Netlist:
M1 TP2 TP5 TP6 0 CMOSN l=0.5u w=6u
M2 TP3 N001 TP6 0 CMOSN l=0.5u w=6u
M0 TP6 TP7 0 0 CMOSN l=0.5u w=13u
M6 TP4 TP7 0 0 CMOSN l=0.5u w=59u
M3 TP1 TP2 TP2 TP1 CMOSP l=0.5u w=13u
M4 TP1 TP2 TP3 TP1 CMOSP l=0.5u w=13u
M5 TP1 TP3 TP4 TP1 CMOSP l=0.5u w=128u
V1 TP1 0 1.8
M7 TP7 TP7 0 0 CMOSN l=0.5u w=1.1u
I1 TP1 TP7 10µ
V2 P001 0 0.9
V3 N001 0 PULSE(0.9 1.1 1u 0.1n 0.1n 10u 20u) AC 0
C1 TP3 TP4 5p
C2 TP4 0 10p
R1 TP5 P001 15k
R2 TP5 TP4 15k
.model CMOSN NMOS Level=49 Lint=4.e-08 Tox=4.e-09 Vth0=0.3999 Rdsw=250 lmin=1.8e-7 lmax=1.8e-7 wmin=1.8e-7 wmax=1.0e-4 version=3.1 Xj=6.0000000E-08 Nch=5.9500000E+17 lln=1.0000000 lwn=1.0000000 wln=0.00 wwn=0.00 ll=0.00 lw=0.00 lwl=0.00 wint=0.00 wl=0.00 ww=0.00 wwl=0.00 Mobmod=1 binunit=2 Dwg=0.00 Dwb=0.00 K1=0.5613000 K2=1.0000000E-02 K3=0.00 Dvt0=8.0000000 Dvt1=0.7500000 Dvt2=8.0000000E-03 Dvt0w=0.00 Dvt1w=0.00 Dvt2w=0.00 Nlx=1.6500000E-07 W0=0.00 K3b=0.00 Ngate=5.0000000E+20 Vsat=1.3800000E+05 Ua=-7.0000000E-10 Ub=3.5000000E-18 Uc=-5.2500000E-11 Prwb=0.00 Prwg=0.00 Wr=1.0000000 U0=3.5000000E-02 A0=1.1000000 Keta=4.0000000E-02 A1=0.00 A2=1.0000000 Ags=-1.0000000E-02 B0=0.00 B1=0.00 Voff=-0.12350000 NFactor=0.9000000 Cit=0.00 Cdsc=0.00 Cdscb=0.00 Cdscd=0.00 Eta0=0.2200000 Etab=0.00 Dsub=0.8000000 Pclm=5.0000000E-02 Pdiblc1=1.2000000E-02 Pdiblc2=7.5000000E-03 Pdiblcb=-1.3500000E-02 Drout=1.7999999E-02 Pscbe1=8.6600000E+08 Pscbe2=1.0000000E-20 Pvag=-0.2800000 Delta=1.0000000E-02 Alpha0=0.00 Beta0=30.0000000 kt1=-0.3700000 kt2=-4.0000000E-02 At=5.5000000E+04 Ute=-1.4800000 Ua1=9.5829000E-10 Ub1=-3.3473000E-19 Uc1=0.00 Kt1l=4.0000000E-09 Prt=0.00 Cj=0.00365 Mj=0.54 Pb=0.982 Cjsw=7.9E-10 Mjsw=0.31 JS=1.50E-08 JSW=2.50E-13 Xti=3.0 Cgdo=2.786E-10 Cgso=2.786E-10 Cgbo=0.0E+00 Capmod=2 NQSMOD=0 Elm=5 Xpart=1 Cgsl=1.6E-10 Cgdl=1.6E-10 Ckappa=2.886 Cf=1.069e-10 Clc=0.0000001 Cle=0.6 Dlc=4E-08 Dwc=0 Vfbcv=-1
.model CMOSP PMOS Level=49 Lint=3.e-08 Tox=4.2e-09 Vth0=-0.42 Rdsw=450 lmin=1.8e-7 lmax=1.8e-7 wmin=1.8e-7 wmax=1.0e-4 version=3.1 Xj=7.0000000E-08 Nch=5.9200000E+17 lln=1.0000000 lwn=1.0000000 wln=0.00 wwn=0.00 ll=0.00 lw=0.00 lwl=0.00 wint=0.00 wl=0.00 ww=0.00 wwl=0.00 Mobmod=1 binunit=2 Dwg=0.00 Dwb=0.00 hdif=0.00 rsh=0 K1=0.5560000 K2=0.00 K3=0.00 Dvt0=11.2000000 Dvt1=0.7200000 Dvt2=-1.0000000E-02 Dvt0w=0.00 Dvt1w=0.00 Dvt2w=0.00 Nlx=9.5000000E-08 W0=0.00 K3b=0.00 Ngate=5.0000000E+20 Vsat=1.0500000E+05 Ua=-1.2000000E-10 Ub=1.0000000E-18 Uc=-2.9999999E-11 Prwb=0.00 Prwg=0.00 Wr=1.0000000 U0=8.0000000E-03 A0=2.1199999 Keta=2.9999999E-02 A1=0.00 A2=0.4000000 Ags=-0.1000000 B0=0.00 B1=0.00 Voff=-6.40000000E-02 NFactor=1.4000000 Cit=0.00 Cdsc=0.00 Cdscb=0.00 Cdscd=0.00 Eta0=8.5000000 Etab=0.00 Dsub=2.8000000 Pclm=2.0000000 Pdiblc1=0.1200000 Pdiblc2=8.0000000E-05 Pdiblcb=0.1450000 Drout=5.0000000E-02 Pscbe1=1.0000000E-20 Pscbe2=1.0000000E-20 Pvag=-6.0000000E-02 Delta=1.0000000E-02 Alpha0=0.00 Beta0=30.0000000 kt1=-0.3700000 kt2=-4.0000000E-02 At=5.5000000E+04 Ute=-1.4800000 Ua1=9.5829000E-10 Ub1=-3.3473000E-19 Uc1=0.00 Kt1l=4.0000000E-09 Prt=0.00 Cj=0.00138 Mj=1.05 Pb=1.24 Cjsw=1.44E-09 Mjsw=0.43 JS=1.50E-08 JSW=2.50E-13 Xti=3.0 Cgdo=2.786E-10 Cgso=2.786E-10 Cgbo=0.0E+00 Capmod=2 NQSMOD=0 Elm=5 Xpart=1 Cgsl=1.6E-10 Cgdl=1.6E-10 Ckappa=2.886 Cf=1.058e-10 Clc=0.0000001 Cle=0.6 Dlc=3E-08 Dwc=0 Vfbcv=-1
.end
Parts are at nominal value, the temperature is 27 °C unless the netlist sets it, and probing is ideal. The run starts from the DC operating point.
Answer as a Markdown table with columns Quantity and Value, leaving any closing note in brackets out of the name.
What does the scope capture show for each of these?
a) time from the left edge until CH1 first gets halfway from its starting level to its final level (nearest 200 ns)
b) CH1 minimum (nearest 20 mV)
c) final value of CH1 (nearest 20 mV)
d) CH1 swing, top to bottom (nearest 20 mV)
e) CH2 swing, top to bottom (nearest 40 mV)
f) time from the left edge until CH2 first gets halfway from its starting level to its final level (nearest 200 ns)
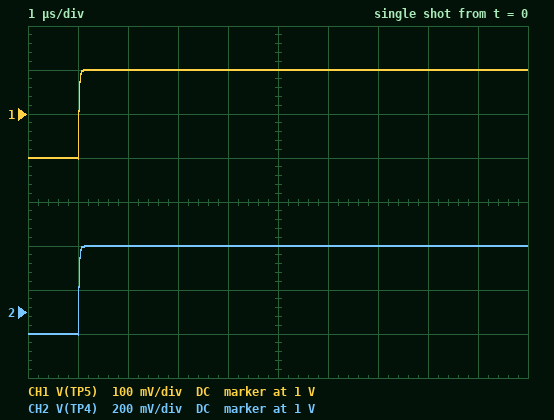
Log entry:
| Quantity | Value |
|---|---|
| time from the left edge until CH1 first gets halfway from its starting level to its final level | 1.0 µs |
| CH1 minimum | 900 mV |
| final value of CH1 | 1.10 V |
| CH1 swing, top to bottom | 200 mV |
| CH2 swing, top to bottom | 400 mV |
| time from the left edge until CH2 first gets halfway from its starting level to its final level | 1.0 µs |
